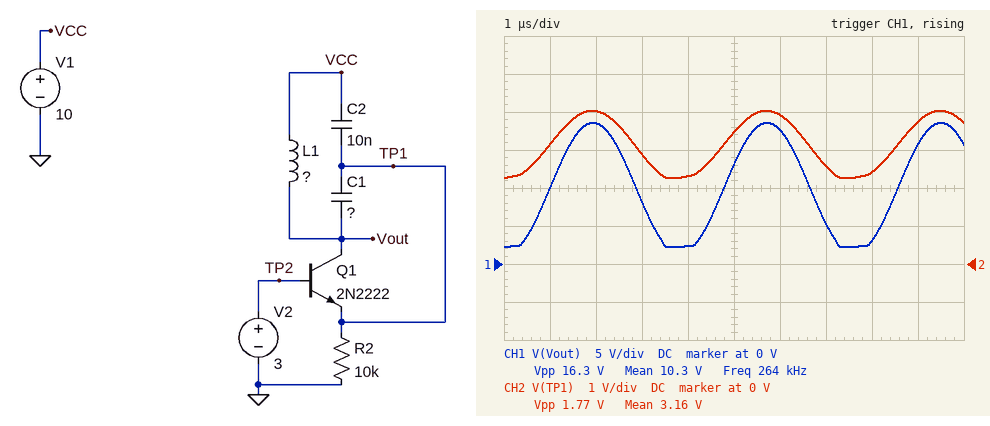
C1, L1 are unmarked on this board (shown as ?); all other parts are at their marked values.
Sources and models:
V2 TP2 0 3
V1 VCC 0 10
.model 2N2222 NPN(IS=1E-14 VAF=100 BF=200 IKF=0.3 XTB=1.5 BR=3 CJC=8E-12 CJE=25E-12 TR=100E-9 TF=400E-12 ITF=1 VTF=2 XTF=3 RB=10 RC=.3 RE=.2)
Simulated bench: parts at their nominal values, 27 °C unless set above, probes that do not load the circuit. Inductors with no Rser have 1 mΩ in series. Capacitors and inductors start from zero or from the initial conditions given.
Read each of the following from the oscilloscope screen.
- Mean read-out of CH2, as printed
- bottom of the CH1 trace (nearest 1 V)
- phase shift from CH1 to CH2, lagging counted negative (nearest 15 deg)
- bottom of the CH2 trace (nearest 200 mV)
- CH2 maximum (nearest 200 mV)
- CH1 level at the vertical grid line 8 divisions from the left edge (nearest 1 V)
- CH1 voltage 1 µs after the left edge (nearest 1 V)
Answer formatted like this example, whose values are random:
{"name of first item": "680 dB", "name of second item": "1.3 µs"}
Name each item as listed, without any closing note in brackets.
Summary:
{"Mean read-out of CH2, as printed": "3.16 V", "bottom of the CH1 trace": "2 V", "phase shift from CH1 to CH2, lagging counted negative": "0 deg", "bottom of the CH2 trace": "2.2 V", "CH2 maximum": "4.0 V", "CH1 level at the vertical grid line 8 divisions from the left edge": "3 V", "CH1 voltage 1 µs after the left edge": "10 V"}
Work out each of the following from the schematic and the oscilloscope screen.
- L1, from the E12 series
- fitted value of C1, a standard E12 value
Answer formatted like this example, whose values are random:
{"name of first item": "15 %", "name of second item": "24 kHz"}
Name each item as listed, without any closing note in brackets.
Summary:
{"L1, from the E12 series": "330 µH", "fitted value of C1, a standard E12 value": "1.2 nF"}
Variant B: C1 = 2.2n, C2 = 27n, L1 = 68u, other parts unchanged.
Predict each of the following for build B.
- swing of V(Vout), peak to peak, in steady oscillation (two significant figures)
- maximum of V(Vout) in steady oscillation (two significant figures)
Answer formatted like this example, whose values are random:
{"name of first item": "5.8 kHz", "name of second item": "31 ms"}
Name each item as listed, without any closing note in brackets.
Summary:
{"swing of V(Vout), peak to peak, in steady oscillation": "48 mV", "maximum of V(Vout) in steady oscillation": "10 V"}
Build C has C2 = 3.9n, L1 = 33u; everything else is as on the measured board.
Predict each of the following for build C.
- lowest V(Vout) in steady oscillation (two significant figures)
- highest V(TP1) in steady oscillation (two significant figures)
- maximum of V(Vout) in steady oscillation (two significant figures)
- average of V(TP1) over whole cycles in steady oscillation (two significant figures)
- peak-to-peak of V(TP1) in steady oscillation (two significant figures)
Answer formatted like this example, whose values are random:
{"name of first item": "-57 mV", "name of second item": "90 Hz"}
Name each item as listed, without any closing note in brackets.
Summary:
{"lowest V(Vout) in steady oscillation": "2.2 V", "highest V(TP1) in steady oscillation": "6.2 V", "maximum of V(Vout) in steady oscillation": "19 V", "average of V(TP1) over whole cycles in steady oscillation": "4.1 V", "peak-to-peak of V(TP1) in steady oscillation": "3.9 V"}
